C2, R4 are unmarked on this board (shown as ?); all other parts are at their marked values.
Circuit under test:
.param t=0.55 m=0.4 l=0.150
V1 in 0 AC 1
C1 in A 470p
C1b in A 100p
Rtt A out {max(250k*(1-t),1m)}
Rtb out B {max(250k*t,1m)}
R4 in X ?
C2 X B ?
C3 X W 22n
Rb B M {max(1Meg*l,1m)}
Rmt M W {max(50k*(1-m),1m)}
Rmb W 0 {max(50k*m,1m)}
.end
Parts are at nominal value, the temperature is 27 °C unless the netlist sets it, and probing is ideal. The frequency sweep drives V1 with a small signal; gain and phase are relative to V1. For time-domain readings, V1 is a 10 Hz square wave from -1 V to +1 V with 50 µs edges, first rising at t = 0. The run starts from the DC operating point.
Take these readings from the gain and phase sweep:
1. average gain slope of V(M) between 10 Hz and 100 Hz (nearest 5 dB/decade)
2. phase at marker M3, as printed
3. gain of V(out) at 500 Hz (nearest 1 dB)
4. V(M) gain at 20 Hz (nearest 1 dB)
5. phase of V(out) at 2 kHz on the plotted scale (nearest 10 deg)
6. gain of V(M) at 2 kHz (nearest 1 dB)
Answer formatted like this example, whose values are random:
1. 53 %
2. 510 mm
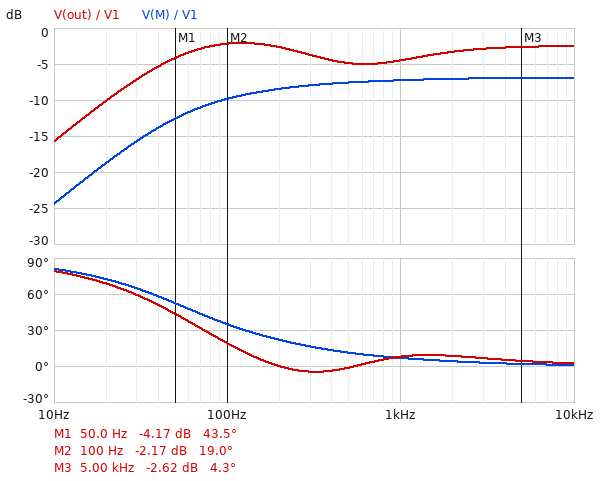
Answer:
1. 15 dB/decade
2. 4.3 deg
3. -5 dB
4. -19 dB
5. 10 deg
6. -7 dB
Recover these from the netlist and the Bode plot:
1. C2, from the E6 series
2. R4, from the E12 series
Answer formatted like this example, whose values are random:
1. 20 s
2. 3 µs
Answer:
1. 10 nF
2. 27 kΩ
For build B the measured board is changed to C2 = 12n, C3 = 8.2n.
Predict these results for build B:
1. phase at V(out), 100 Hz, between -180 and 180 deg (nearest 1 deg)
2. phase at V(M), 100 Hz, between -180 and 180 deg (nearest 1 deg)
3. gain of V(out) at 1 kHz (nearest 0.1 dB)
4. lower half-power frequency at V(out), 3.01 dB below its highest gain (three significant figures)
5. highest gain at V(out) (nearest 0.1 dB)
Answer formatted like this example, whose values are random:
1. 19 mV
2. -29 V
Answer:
1. 24 deg
2. 35 deg
3. -4.0 dB
4. 45.9 Hz
5. -1.3 dB
